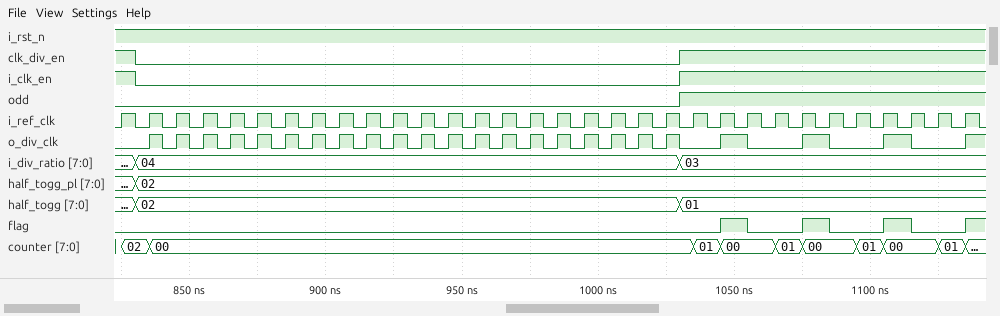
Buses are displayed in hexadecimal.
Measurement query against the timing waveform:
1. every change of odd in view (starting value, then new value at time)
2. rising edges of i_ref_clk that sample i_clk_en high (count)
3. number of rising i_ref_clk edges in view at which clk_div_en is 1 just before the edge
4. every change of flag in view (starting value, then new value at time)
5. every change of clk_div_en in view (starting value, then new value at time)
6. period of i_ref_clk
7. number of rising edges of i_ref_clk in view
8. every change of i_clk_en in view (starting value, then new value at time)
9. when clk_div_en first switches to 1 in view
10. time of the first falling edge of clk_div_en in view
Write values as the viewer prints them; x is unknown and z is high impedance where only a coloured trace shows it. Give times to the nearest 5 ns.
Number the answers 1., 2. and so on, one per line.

1. 0, 1 at 1030 ns
2. 12
3. 12
4. 0, 1 at 1045 ns, 0 at 1055 ns, 1 at 1075 ns, 0 at 1085 ns, 1 at 1105 ns, 0 at 1115 ns, 1 at 1135 ns
5. 1, 0 at 830 ns, 1 at 1030 ns
6. 10 ns
7. 32
8. 1, 0 at 830 ns, 1 at 1030 ns
9. 1030 ns
10. 830 ns
